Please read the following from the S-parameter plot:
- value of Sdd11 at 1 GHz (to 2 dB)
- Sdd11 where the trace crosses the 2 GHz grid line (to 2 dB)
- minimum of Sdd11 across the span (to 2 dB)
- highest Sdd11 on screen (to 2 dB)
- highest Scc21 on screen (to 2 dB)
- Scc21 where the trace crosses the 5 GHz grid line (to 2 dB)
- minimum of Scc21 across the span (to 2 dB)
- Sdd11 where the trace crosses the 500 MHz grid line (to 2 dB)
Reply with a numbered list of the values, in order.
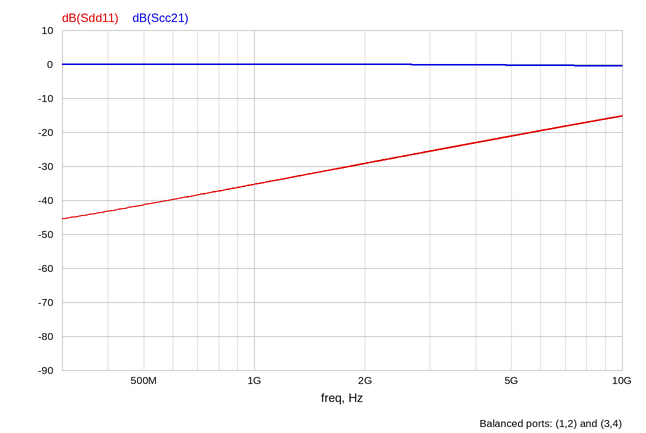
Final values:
1. -36 dB
2. -30 dB
3. -46 dB
4. -16 dB
5. 0 dB
6. 0 dB
7. 0 dB
8. -42 dB
